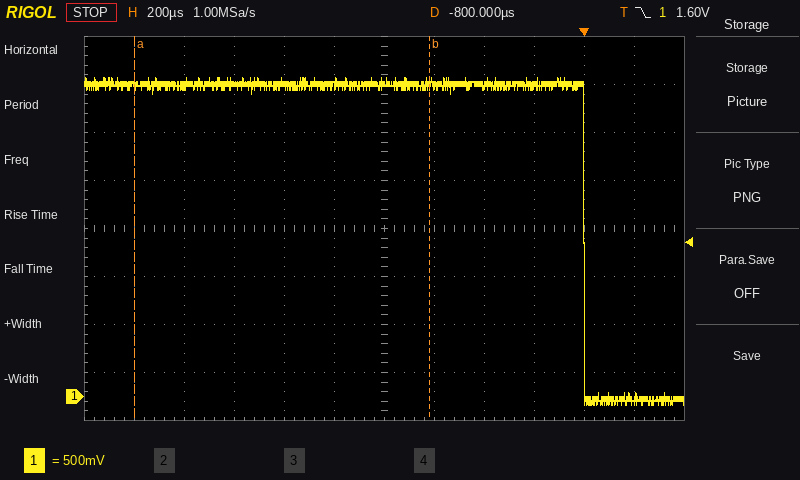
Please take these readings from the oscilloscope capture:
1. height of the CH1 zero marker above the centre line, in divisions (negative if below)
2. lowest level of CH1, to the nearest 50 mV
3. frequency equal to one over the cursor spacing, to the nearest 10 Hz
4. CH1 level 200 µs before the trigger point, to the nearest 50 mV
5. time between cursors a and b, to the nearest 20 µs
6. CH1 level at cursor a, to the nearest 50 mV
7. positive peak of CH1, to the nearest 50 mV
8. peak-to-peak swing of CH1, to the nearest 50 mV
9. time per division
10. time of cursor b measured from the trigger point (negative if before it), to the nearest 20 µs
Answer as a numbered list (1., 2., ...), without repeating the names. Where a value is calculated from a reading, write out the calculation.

1. -3.5 div
2. -100 mV
3. 1 / 1.18 ms ≈ 850 Hz
4. 3.25 V
5. 1.18 ms
6. 3.25 V
7. 3.30 V
8. 3.30 V − (-100 mV) = 3.40 V
9. 200 µs
10. -620 µs
